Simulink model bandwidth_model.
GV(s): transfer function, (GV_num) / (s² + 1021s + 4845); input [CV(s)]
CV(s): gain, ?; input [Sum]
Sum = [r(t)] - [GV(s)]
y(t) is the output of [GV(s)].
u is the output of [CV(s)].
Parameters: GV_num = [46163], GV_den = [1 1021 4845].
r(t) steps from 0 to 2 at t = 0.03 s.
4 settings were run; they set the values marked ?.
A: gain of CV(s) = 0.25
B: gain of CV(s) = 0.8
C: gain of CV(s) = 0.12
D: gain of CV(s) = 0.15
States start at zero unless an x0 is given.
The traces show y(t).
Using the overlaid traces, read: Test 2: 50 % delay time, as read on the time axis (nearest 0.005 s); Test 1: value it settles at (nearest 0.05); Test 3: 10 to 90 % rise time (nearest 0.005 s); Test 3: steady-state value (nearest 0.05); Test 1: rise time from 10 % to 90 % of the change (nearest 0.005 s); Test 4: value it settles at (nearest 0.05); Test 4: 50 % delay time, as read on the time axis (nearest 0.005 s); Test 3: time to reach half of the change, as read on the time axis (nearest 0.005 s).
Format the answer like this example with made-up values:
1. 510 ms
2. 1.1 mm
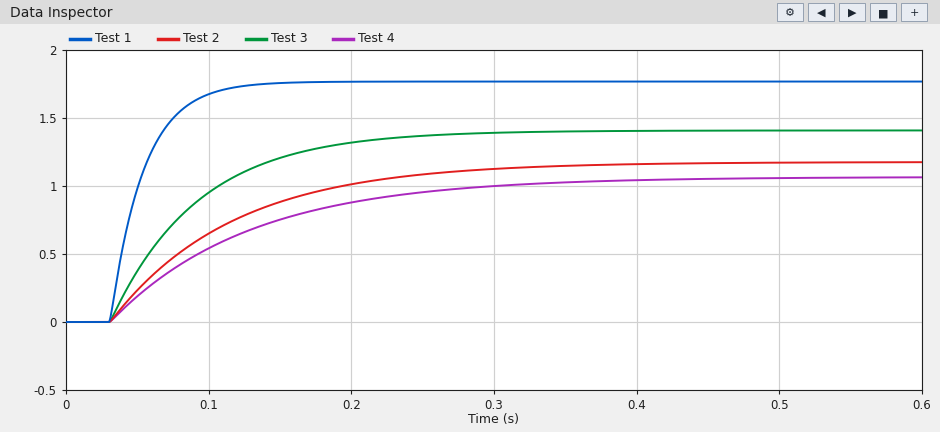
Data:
1. 0.090 s
2. 1.75
3. 0.135 s
4. 1.40
5. 0.050 s
6. 1.05
7. 0.100 s
8. 0.075 s
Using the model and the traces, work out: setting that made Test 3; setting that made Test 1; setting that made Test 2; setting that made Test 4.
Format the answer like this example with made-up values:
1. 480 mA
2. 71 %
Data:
1. A
2. B
3. D
4. C
